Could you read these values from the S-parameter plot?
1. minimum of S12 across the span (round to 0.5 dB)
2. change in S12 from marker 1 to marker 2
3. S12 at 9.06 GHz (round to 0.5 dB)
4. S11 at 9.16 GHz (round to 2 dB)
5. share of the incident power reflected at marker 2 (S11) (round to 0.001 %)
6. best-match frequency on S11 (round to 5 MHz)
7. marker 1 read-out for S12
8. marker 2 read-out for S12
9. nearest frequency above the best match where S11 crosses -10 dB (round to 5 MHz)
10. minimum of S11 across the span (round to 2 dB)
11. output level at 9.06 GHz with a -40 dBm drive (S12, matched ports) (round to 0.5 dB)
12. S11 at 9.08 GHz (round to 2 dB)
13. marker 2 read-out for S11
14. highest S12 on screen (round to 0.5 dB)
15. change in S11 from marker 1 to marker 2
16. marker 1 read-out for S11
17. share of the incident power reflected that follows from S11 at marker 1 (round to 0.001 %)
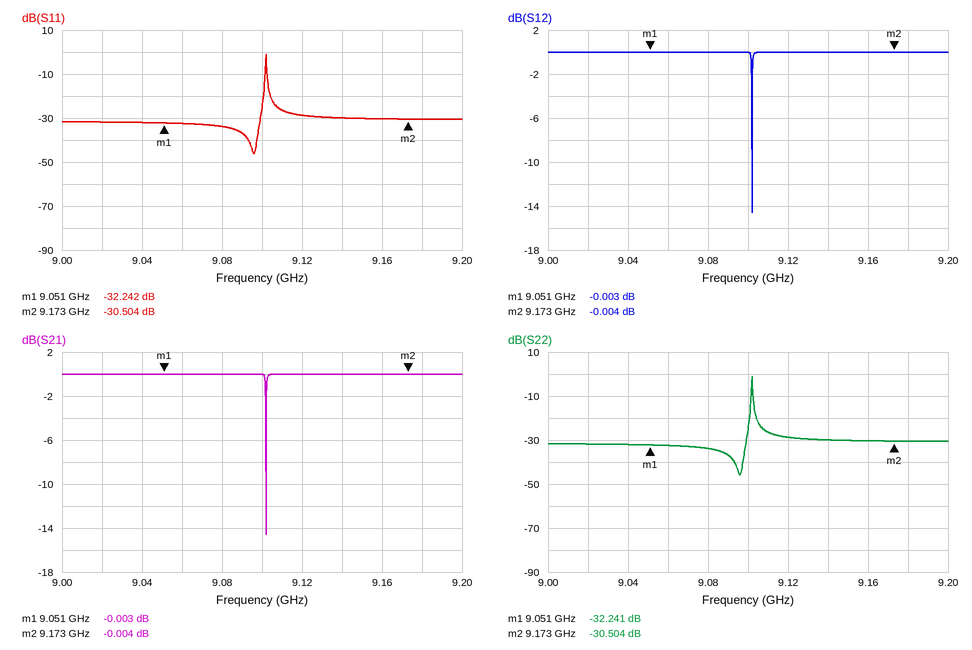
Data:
-14.5 dB
-0.001 dB
0.0 dB
-30 dB
0.089 %
9.095 GHz
-0.003 dB
-0.004 dB
9.100 GHz
-46 dB
-40.0 dBm
-34 dB
-30.504 dB
0.0 dB
1.738 dB
-32.242 dB
0.060 %
